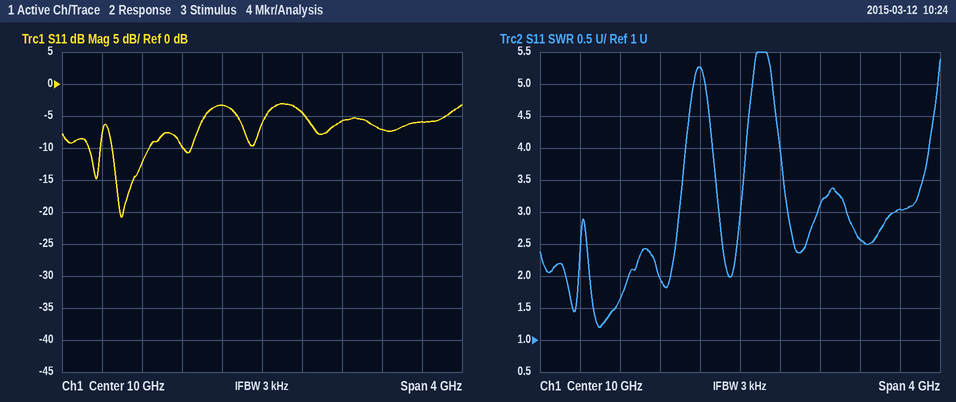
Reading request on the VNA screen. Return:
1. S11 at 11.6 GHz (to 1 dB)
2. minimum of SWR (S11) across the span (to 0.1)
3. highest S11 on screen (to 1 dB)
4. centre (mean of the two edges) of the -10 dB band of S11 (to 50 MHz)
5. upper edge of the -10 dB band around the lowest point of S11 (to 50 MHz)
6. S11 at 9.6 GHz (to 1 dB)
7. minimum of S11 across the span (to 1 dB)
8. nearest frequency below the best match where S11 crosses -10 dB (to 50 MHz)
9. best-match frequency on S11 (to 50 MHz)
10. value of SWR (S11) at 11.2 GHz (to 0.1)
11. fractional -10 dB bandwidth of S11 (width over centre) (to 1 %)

-6 dB
1.2
-3 dB
8.70 GHz
8.85 GHz
-3 dB
-21 dB
8.50 GHz
8.60 GHz
2.6
4 %
